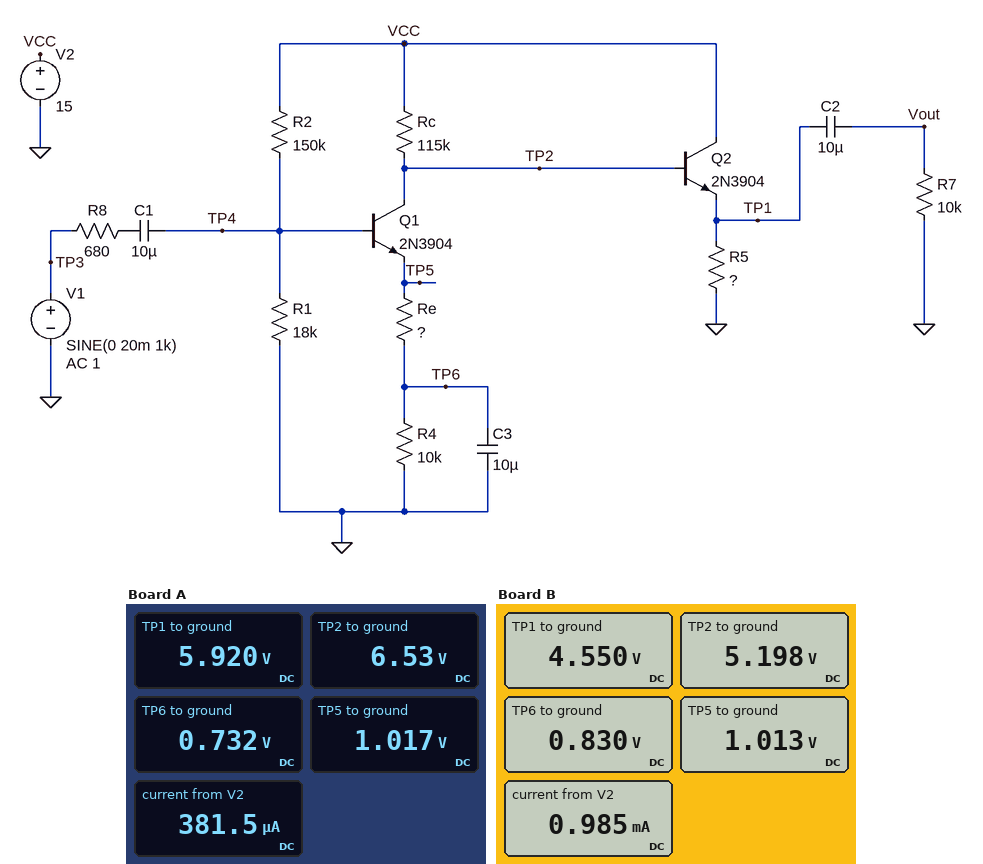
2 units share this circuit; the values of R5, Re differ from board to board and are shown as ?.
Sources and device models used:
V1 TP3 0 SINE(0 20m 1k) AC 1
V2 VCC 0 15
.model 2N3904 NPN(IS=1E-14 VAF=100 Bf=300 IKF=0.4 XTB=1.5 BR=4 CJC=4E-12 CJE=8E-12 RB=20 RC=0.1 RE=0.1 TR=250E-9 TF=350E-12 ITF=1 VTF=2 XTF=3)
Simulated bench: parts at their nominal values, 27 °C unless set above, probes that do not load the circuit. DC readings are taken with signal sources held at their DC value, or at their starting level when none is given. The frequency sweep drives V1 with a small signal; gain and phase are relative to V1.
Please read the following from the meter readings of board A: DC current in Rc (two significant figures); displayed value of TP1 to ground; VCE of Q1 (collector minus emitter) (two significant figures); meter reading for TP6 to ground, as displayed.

74 µA
5.920 V
5.5 V
0.732 V
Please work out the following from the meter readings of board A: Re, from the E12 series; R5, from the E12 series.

3.9 kΩ
27 kΩ
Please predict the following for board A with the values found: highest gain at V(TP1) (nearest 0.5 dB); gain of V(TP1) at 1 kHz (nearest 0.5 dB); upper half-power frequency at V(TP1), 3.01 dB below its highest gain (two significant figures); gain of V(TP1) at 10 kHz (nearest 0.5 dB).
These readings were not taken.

27.5 dB
27.5 dB
330 kHz
27.5 dB
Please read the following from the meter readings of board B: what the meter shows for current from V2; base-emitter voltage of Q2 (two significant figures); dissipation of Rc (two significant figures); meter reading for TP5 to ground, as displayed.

0.985 mA
650 mV
840 µW
1.013 V
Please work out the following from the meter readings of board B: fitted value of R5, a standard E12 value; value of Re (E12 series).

5.6 kΩ
2.2 kΩ
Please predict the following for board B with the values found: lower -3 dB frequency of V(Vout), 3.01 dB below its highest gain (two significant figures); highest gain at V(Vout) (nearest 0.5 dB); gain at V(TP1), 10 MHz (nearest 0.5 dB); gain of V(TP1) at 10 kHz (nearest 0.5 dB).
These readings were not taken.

8.0 Hz
32.0 dB
3.0 dB
32.0 dB
